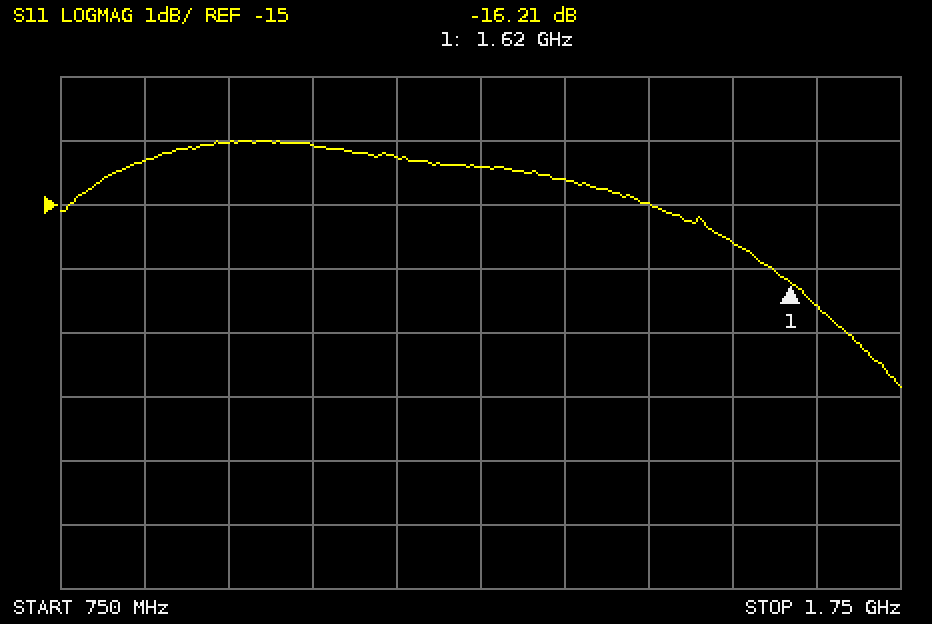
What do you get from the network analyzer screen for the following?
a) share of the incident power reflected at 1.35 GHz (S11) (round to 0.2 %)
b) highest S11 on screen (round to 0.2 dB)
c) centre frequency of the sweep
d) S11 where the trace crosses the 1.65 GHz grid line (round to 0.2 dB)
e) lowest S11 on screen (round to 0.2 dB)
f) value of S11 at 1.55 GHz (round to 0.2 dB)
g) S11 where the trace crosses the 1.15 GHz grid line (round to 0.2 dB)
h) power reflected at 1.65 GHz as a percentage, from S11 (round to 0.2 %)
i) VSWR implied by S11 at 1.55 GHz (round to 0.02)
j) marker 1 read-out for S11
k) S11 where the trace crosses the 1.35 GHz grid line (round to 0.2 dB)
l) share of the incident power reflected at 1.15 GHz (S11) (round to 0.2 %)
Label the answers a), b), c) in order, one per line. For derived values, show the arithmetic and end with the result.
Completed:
a) 10^(-14.6/10) ≈ 3.47 %, so 3.4 % to the nearest 0.2 %
b) -14.0 dB
c) 1.25 GHz
d) -16.6 dB
e) -17.8 dB
f) -15.6 dB
g) -14.2 dB
h) 10^(-16.6/10) ≈ 2.2 %
i) |Γ| = 10^(-15.6/20) = 0.1660; VSWR = (1 + 0.1660)/(1 − 0.1660) ≈ 1.40
j) -16.21 dB
k) -14.6 dB
l) 10^(-14.2/10) ≈ 3.8 %
